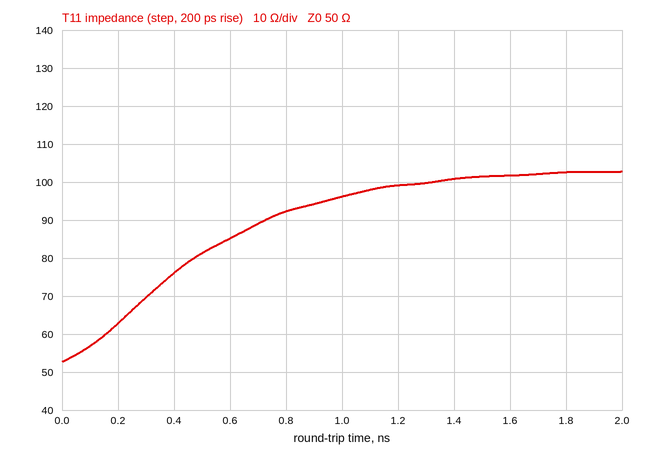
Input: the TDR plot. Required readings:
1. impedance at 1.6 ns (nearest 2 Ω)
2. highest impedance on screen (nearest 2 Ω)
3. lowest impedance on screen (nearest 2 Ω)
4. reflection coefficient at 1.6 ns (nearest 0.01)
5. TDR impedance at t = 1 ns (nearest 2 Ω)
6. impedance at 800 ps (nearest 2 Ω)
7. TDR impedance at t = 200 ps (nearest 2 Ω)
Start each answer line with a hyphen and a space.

- 102 Ω
- 102 Ω
- 52 Ω
- +0.34
- 96 Ω
- 92 Ω
- 62 Ω
